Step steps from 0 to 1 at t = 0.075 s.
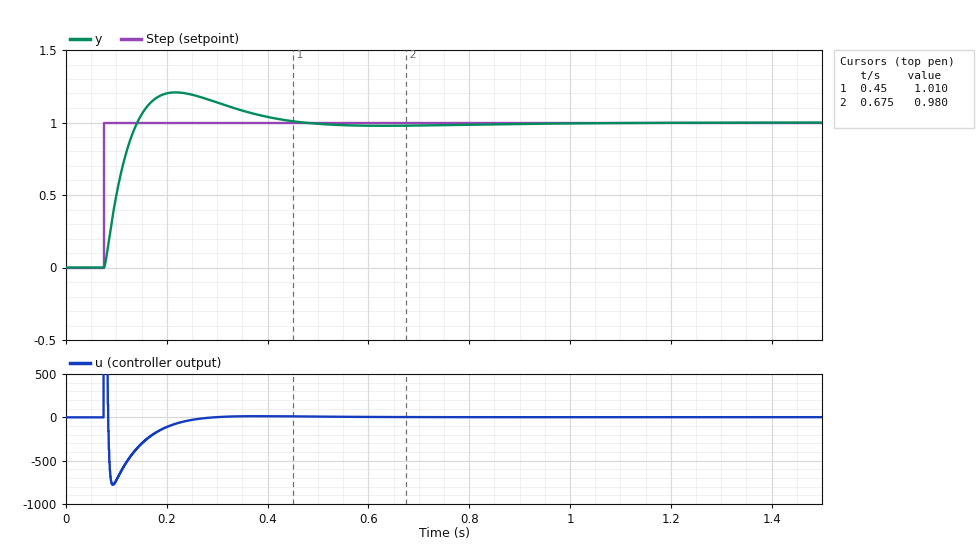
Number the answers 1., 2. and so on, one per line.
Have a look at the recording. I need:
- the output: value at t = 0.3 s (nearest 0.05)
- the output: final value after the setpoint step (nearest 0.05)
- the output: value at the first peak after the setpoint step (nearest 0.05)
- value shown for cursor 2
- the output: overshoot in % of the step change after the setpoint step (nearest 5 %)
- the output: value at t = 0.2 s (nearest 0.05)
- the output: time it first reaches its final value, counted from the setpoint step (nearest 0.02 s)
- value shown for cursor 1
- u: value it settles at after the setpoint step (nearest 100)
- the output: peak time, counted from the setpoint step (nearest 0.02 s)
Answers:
1. 1.15
2. 1.00
3. 1.20
4. 0.980
5. 20 %
6. 1.20
7. 0.06 s
8. 1.010
9. 0
10. 0.14 s
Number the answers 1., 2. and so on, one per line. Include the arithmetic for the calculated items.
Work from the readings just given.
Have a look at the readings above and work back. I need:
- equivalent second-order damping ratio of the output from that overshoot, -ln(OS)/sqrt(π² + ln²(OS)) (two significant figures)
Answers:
1. ln(0.2) = -1.609; 1.609 / sqrt(9.870 + 2.590) = 0.46
